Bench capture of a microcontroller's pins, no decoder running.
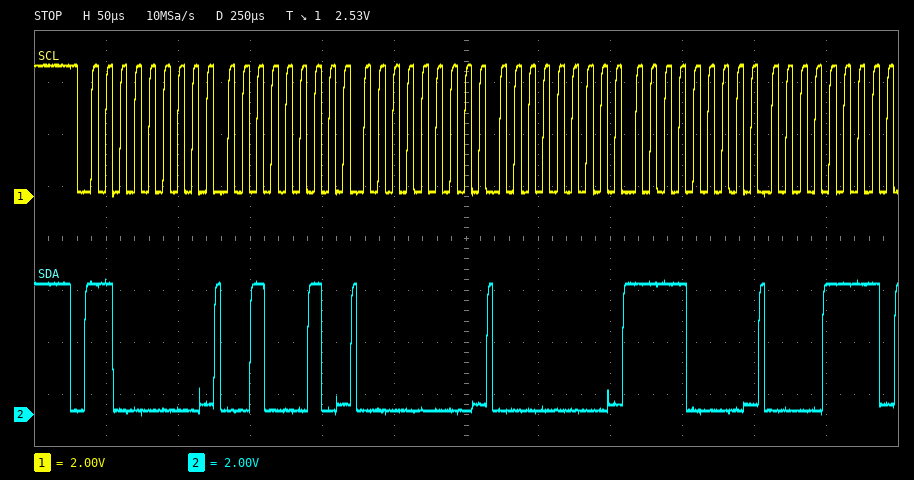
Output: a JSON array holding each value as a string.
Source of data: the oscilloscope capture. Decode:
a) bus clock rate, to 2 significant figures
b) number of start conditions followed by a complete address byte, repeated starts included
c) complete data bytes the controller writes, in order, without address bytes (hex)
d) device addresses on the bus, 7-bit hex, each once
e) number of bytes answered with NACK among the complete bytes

["100 kHz", "1", "22 00 00 F0 0F", "0x60", "0"]
